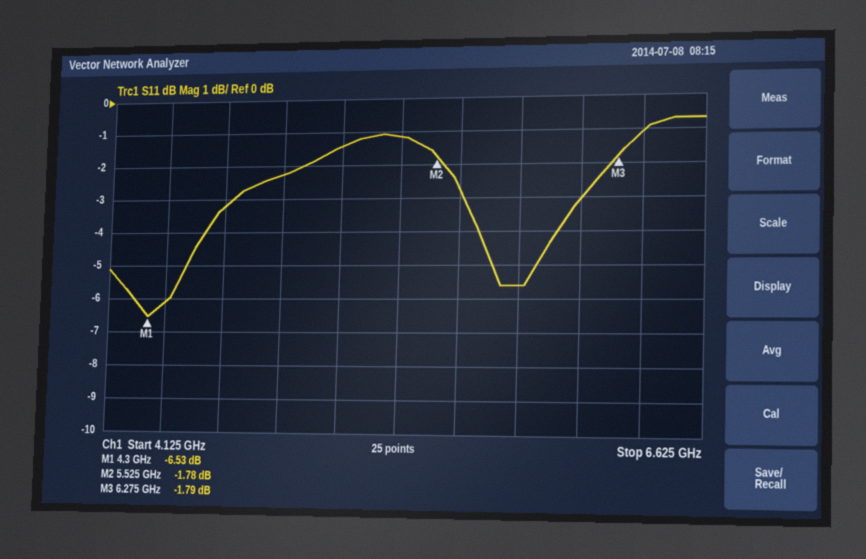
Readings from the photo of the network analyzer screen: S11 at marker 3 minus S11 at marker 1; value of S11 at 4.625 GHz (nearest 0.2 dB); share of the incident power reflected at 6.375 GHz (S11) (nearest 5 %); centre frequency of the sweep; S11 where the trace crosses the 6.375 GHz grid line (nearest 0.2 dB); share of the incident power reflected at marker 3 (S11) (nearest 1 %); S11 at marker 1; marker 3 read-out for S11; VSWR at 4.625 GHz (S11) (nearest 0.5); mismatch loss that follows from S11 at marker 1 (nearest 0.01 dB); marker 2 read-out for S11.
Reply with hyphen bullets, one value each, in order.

- 4.74 dB
- -3.2 dB
- 80 %
- 5.375 GHz
- -1.0 dB
- 66 %
- -6.53 dB
- -1.79 dB
- 5.5
- 1.09 dB
- -1.78 dB
